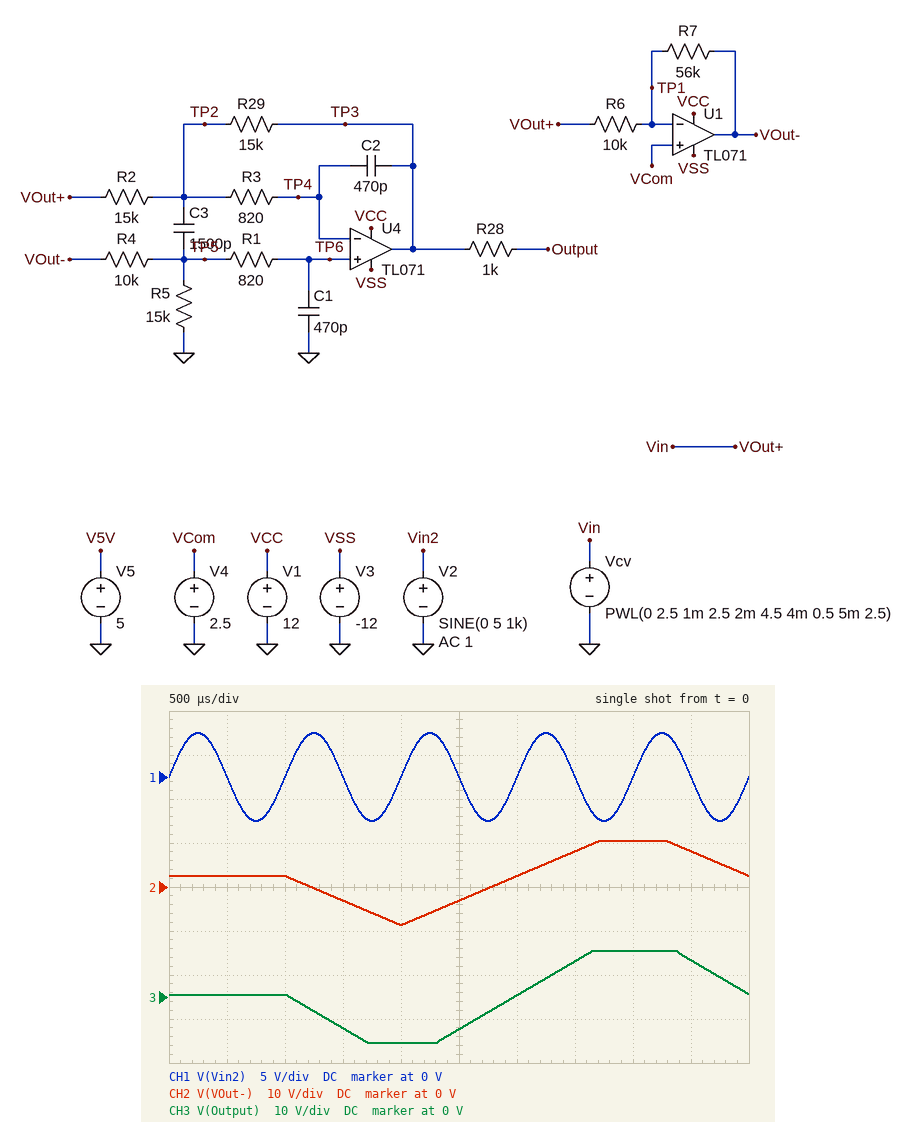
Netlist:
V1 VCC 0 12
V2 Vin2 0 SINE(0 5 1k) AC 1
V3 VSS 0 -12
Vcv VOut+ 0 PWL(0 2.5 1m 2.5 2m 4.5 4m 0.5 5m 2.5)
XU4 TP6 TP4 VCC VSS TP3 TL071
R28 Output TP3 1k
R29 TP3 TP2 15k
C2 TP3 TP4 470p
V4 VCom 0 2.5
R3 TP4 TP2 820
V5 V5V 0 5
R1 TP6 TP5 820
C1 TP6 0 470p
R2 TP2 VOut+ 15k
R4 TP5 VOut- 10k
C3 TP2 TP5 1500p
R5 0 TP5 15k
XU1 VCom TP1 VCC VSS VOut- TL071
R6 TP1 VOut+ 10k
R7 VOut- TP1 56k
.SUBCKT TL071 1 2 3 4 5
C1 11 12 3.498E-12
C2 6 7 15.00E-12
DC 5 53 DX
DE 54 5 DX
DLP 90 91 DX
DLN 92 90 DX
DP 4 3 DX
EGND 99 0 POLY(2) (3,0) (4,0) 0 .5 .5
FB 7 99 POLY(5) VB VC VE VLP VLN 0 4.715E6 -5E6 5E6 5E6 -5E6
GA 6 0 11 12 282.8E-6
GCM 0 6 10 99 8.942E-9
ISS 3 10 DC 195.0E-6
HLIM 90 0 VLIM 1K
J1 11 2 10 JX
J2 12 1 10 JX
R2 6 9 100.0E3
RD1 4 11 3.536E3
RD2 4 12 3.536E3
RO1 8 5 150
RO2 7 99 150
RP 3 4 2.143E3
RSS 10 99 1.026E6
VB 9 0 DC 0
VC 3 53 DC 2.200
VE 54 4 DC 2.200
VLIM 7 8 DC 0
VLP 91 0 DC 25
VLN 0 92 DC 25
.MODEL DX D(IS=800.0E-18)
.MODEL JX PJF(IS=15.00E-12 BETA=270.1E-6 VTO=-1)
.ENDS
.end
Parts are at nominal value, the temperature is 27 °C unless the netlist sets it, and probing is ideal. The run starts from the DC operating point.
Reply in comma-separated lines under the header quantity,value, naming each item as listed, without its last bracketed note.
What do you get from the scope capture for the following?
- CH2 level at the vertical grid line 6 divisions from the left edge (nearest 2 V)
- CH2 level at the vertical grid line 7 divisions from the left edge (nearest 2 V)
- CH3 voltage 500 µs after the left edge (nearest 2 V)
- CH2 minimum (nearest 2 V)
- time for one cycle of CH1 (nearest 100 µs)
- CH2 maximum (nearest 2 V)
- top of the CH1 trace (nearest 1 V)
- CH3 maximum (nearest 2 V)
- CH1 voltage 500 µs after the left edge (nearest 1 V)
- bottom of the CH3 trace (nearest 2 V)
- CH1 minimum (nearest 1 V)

quantity,value
CH2 level at the vertical grid line 6 divisions from the left edge,2 V
CH2 level at the vertical grid line 7 divisions from the left edge,8 V
CH3 voltage 500 µs after the left edge,0 V
CH2 minimum,-8 V
time for one cycle of CH1,1.0 ms
CH2 maximum,10 V
top of the CH1 trace,5 V
CH3 maximum,10 V
CH1 voltage 500 µs after the left edge,0 V
bottom of the CH3 trace,-10 V
CH1 minimum,-5 V
